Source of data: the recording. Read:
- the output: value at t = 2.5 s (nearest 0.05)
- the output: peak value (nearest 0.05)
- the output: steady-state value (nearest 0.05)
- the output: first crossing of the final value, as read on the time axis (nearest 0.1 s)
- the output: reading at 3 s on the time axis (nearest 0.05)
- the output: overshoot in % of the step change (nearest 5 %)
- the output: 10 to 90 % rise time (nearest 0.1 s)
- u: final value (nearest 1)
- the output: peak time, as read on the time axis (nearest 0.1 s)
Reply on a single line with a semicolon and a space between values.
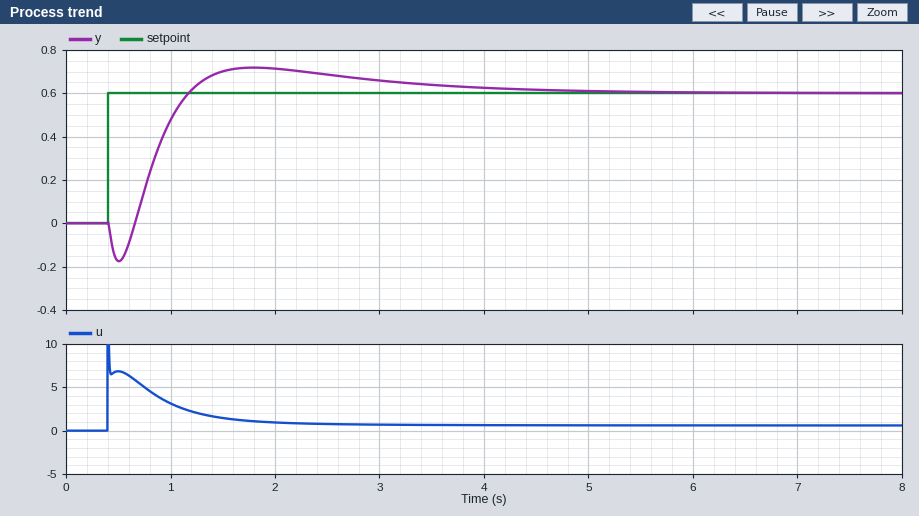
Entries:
0.70; 0.70; 0.60; 1.2 s; 0.65; 20 %; 0.4 s; 1; 1.8 s
